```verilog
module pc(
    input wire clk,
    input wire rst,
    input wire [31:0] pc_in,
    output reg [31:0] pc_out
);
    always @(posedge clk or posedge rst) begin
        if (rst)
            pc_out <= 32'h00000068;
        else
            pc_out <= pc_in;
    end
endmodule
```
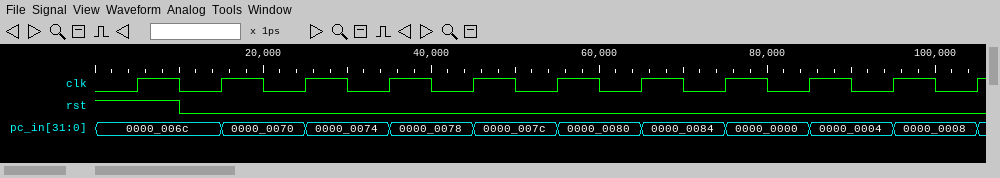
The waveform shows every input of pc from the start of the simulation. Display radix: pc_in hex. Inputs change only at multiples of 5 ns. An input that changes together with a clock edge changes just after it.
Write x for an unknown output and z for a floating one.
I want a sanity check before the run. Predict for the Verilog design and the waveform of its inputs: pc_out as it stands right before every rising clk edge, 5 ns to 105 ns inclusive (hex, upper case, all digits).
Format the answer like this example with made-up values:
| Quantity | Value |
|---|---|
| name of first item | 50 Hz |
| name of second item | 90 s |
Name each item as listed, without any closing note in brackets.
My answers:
| Quantity | Value |
|---|---|
| pc_out as it stands right before every rising clk edge, 5 ns to 105 ns inclusive | 00000068, 00000068, 0000006C, 00000070, 00000074, 00000078, 0000007C, 00000080, 00000084, 00000000, 00000004 |
